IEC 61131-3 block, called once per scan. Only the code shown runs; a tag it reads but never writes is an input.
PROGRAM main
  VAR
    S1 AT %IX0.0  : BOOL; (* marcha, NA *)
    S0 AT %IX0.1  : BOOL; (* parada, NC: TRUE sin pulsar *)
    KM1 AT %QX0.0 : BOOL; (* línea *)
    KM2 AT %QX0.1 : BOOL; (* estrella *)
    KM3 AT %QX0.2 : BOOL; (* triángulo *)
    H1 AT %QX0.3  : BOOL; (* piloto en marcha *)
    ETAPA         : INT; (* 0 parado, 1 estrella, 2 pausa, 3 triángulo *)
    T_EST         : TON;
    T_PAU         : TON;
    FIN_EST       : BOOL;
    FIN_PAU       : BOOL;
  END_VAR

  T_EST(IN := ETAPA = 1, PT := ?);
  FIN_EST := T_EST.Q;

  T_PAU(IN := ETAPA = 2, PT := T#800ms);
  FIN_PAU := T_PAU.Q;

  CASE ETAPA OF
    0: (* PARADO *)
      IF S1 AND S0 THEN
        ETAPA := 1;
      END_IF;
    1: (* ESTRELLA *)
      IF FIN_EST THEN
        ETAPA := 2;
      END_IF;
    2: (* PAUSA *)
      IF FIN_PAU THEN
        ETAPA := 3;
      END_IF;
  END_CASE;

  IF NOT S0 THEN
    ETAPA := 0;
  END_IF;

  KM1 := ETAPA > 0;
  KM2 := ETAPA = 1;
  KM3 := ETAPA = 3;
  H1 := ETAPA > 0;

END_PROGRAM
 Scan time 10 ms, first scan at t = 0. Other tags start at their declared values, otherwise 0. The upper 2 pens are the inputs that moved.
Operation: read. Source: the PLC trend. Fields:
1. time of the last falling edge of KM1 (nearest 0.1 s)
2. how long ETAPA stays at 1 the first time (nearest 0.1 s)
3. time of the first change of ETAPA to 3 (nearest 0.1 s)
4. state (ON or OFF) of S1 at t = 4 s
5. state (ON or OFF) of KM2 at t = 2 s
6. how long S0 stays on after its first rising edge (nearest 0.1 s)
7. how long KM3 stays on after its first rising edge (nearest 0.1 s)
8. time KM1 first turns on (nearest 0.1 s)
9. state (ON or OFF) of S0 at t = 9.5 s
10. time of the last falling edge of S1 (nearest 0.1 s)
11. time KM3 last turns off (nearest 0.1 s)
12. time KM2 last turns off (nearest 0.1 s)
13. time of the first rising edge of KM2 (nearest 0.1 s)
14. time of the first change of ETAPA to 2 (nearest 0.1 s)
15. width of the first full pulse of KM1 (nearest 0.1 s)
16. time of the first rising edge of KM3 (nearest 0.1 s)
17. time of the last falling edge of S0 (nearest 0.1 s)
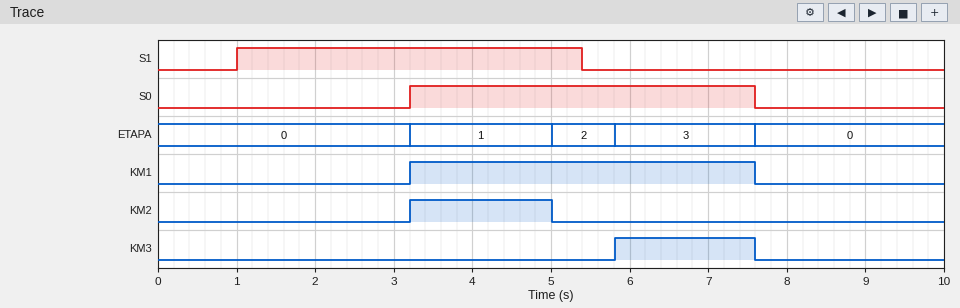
7.6 s
1.8 s
5.8 s
ON
OFF
4.4 s
1.8 s
3.2 s
OFF
5.4 s
7.6 s
5.0 s
3.2 s
5.0 s
4.4 s
5.8 s
7.6 s
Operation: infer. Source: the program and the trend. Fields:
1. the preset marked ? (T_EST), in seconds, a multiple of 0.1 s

1.8 s
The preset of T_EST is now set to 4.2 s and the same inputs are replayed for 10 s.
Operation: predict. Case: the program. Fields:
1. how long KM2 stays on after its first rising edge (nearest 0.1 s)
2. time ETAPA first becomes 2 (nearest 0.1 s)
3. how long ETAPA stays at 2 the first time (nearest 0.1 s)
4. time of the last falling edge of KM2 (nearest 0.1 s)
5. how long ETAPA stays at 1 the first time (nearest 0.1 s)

4.2 s
7.4 s
0.2 s
7.4 s
4.2 s
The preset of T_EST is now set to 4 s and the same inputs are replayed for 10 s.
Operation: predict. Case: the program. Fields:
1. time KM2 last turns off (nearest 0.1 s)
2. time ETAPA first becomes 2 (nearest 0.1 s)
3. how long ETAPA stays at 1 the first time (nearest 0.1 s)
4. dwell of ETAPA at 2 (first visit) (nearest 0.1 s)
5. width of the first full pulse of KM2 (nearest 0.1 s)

7.2 s
7.2 s
4.0 s
0.4 s
4.0 s
